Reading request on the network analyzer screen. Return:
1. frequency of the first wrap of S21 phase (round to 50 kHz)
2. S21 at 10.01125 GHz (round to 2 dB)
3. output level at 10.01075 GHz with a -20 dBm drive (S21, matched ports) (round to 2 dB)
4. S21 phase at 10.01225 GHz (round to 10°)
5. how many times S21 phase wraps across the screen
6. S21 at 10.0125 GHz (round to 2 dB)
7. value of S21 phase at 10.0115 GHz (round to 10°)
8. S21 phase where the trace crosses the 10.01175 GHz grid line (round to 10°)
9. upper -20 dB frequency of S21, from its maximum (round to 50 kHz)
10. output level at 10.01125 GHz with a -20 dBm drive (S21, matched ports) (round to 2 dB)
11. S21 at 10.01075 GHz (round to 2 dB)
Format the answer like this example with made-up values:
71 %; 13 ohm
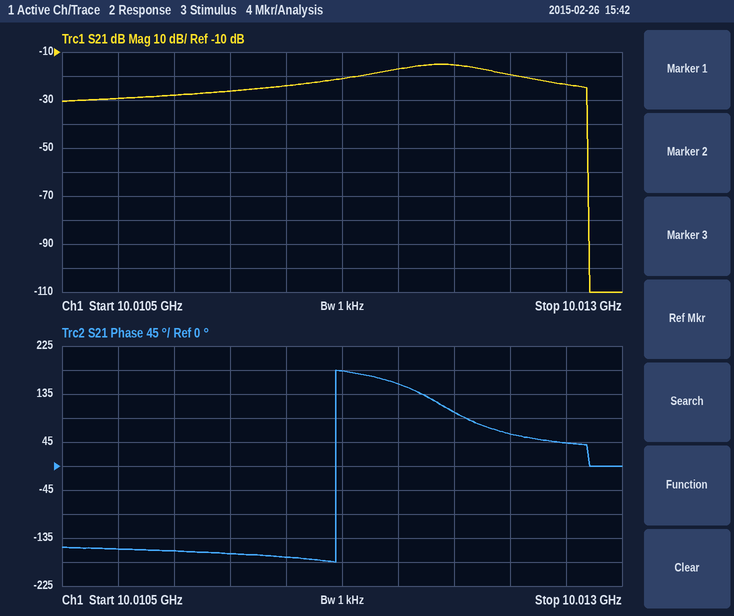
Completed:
10.01170 GHz; -26 dB; -50 dBm; 100°; 1; -20 dB; -170°; 180°; 10.01285 GHz; -46 dBm; -30 dB
